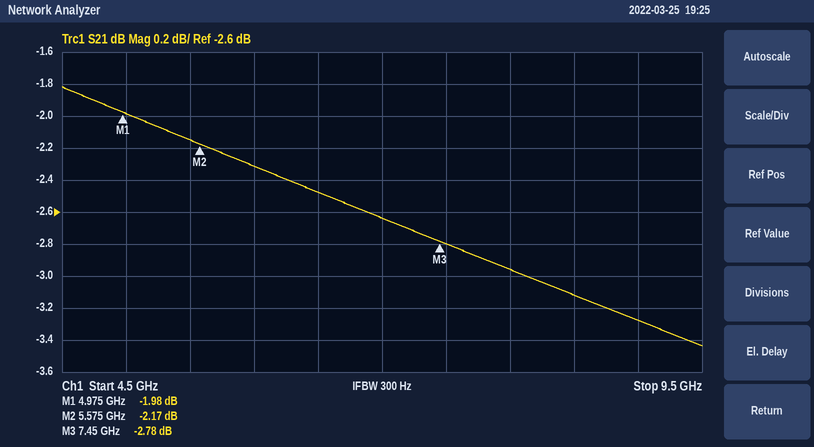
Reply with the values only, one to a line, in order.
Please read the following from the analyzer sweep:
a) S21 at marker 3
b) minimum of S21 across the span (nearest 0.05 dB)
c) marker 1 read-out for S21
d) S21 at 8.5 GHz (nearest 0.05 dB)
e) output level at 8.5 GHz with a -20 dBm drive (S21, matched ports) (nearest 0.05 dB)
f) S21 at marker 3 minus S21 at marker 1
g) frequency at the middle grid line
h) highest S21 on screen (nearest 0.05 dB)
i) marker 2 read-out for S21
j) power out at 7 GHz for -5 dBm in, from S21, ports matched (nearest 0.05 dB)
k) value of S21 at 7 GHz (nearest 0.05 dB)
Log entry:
-2.78 dB
-3.45 dB
-1.98 dB
-3.10 dB
-23.10 dBm
-0.80 dB
7 GHz
-1.80 dB
-2.17 dB
-7.65 dBm
-2.65 dB
